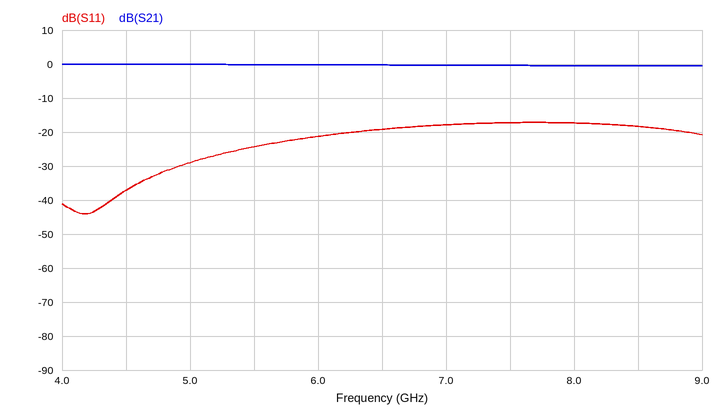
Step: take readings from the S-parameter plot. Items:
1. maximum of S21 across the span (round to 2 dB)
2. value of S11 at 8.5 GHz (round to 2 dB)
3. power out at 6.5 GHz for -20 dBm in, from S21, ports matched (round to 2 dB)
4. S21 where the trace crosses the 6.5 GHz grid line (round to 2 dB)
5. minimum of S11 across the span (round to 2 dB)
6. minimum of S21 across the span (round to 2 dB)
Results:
0 dB
-18 dB
-20 dBm
0 dB
-44 dB
0 dB
